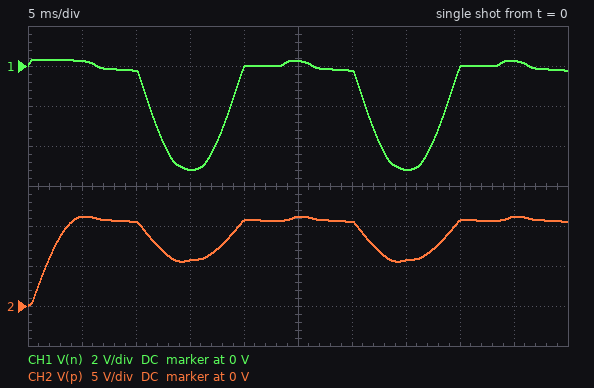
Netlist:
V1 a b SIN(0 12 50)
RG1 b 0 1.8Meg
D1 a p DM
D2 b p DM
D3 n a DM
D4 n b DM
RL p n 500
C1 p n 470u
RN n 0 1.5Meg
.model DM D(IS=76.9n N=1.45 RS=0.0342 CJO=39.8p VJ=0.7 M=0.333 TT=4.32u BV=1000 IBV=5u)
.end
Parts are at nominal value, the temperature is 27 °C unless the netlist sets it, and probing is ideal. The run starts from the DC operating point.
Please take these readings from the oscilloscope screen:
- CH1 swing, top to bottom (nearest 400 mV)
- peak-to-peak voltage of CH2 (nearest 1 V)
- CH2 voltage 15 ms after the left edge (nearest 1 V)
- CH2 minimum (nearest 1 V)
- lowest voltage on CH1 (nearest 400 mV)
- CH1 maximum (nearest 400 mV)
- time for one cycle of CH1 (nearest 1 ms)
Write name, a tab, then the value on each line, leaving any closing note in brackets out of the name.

CH1 swing, top to bottom	5.6 V
peak-to-peak voltage of CH2	11 V
CH2 voltage 15 ms after the left edge	6 V
CH2 minimum	0 V
lowest voltage on CH1	-5.2 V
CH1 maximum	400 mV
time for one cycle of CH1	20 ms
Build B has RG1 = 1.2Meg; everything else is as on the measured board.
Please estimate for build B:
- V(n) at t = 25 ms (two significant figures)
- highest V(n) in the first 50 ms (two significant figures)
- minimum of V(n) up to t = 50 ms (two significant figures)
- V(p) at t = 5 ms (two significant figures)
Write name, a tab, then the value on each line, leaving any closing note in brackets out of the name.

V(n) at t = 25 ms	300 mV
highest V(n) in the first 50 ms	390 mV
minimum of V(n) up to t = 50 ms	-6.4 V
V(p) at t = 5 ms	11 V
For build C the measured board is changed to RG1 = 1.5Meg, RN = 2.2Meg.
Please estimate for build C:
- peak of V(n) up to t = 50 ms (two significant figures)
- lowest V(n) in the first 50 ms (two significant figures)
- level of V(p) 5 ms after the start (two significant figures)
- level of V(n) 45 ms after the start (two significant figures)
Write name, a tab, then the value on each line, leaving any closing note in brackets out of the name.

peak of V(n) up to t = 50 ms	410 mV
lowest V(n) in the first 50 ms	-6.8 V
level of V(p) 5 ms after the start	11 V
level of V(n) 45 ms after the start	320 mV
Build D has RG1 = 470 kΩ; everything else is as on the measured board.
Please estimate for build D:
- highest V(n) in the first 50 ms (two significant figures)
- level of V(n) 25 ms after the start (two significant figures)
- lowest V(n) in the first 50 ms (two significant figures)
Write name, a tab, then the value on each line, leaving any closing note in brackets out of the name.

highest V(n) in the first 50 ms	530 mV
level of V(n) 25 ms after the start	410 mV
lowest V(n) in the first 50 ms	-8.7 V
